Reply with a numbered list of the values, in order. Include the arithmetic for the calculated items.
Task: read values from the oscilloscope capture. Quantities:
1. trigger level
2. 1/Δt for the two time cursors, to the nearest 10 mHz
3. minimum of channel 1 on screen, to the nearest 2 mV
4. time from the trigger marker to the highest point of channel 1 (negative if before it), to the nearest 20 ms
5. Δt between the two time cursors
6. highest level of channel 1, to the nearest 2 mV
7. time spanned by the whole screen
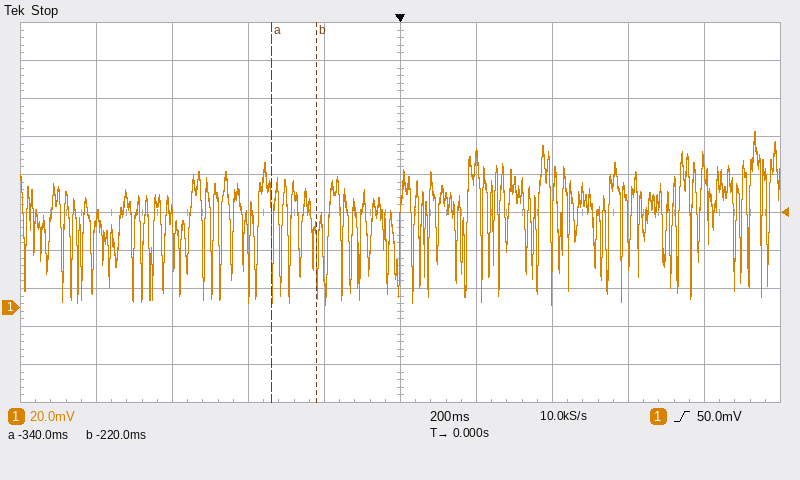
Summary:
1. 50.0 mV
2. 1 / 120 ms ≈ 8.33 Hz
3. 2 mV
4. +940 ms
5. -220 ms − (-340 ms) = 120 ms
6. 92 mV
7. 2 s
